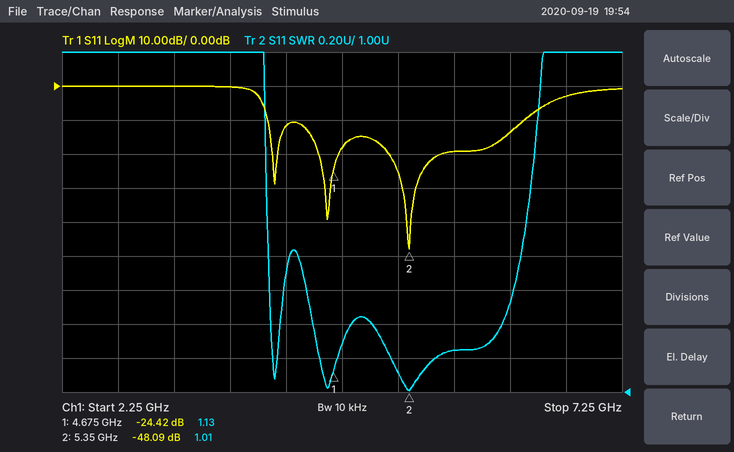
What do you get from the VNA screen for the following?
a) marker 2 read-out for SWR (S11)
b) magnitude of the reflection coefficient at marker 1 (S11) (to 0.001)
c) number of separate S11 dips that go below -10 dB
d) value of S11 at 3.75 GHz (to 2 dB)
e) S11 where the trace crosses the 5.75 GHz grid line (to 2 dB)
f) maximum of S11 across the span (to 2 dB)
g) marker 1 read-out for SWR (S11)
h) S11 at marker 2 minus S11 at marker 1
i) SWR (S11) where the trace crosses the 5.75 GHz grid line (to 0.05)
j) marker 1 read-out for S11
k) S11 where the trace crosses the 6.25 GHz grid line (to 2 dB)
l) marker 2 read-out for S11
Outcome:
1.01
0.060
3
0 dB
-20 dB
0 dB
1.13
-23.67 dB
1.25
-24.42 dB
-14 dB
-48.09 dB
